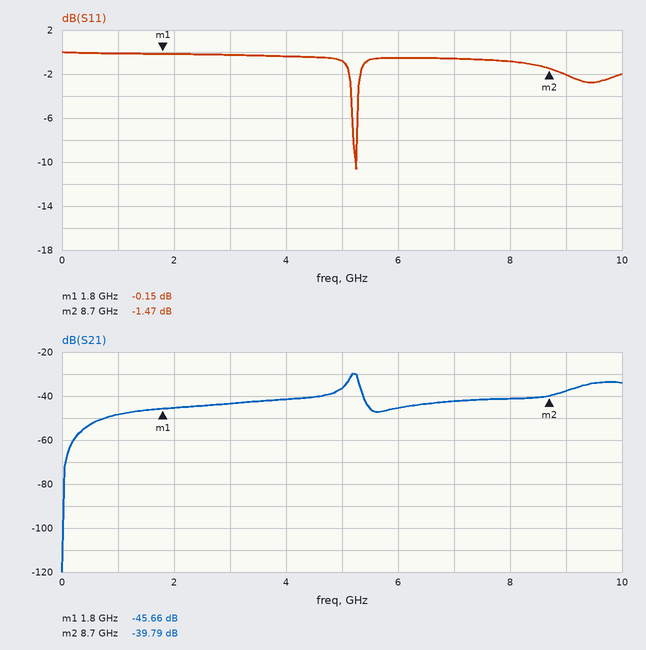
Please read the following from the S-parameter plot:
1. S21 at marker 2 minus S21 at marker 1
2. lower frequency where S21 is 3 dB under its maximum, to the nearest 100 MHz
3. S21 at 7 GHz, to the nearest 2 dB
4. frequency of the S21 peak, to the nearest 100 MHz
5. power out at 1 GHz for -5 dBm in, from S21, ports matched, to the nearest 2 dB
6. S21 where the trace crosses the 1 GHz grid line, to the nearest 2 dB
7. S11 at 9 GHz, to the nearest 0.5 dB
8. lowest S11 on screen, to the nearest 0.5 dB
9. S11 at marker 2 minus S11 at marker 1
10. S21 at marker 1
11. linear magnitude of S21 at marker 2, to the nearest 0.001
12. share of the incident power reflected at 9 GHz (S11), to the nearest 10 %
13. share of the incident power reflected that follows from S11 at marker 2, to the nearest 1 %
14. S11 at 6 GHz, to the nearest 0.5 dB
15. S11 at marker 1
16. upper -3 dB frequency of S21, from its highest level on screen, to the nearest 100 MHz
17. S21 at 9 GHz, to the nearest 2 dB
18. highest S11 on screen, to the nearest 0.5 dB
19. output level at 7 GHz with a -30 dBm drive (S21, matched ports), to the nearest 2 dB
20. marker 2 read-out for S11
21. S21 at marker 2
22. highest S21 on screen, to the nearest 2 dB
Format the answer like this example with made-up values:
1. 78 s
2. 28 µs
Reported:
1. 5.87 dB
2. 5.1 GHz
3. -42 dB
4. 5.2 GHz
5. -54 dBm
6. -48 dB
7. -2.0 dB
8. -10.5 dB
9. -1.32 dB
10. -45.66 dB
11. 0.010
12. 60 %
13. 71 %
14. -0.5 dB
15. -0.15 dB
16. 5.3 GHz
17. -38 dB
18. 0.0 dB
19. -72 dBm
20. -1.47 dB
21. -39.79 dB
22. -30 dB
